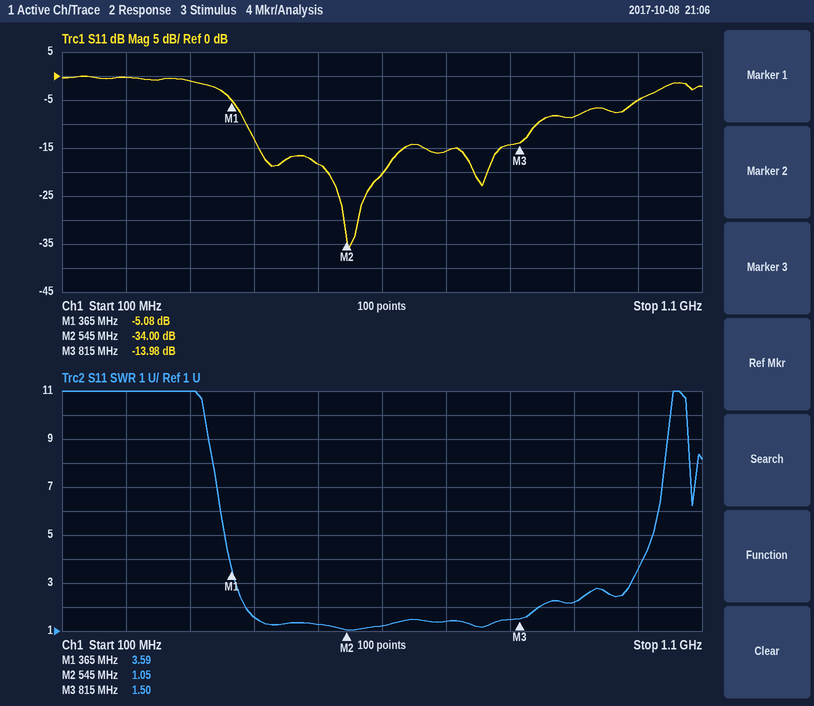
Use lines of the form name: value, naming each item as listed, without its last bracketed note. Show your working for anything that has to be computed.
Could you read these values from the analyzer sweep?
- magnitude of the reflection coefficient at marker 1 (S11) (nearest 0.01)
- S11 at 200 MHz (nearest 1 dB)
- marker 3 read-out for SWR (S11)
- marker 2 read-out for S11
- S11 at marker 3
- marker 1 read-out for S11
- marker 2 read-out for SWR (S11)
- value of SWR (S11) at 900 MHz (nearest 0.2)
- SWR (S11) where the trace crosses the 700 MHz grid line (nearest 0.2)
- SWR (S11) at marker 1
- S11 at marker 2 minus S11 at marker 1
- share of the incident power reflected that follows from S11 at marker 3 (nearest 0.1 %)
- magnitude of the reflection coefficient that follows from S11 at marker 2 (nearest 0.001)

magnitude of the reflection coefficient at marker 1 (S11): 10^(-5.08/20) ≈ 0.56
S11 at 200 MHz: 0 dB
marker 3 read-out for SWR: 1.50
marker 2 read-out for S11: -34.00 dB
S11 at marker 3: -13.98 dB
marker 1 read-out for S11: -5.08 dB
marker 2 read-out for SWR: 1.05
value of SWR (S11) at 900 MHz: 2.2
SWR (S11) where the trace crosses the 700 MHz grid line: 1.4
SWR (S11) at marker 1: 3.59
S11 at marker 2 minus S11 at marker 1: -34 − (-5.08) = -28.92 dB
share of the incident power reflected that follows from S11 at marker 3: 10^(-13.98/10) ≈ 4.0 %
magnitude of the reflection coefficient that follows from S11 at marker 2: 10^(-34/20) ≈ 0.020
